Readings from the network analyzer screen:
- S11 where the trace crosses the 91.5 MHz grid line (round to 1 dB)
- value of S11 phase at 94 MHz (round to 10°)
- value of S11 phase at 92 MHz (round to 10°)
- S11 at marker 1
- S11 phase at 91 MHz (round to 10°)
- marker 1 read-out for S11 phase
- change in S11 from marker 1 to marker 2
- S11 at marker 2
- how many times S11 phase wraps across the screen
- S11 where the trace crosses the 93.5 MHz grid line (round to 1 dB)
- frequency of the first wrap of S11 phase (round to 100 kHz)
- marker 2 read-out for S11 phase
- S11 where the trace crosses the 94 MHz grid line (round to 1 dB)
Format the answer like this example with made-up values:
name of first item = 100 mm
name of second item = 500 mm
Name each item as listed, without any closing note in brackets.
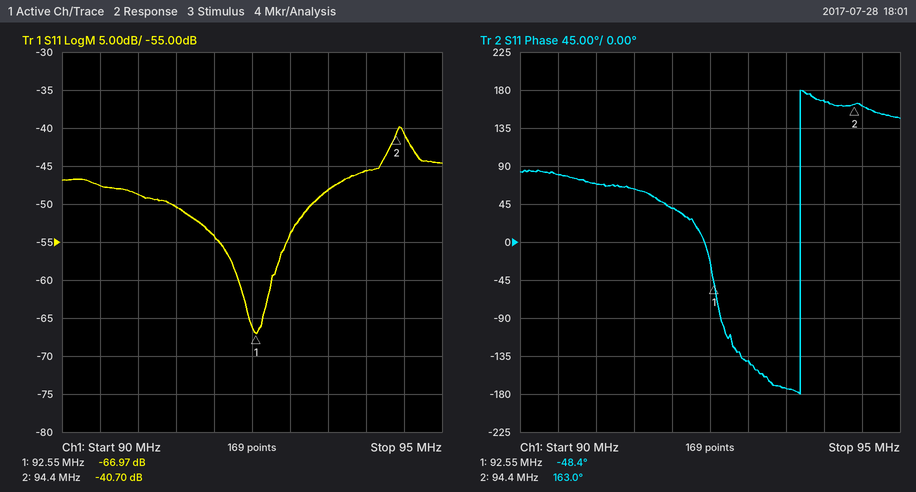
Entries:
S11 where the trace crosses the 91.5 MHz grid line = -50 dB
value of S11 phase at 94 MHz = 170°
value of S11 phase at 92 MHz = 40°
S11 at marker 1 = -66.97 dB
S11 phase at 91 MHz = 70°
marker 1 read-out for S11 phase = -48.4°
change in S11 from marker 1 to marker 2 = 26.27 dB
S11 at marker 2 = -40.70 dB
how many times S11 phase wraps across the screen = 1
S11 where the trace crosses the 93.5 MHz grid line = -48 dB
frequency of the first wrap of S11 phase = 93.7 MHz
marker 2 read-out for S11 phase = 163.0°
S11 where the trace crosses the 94 MHz grid line = -46 dB
